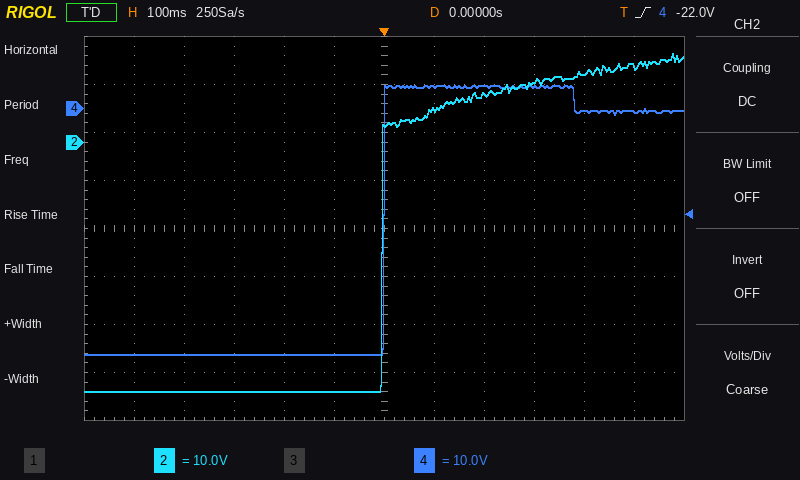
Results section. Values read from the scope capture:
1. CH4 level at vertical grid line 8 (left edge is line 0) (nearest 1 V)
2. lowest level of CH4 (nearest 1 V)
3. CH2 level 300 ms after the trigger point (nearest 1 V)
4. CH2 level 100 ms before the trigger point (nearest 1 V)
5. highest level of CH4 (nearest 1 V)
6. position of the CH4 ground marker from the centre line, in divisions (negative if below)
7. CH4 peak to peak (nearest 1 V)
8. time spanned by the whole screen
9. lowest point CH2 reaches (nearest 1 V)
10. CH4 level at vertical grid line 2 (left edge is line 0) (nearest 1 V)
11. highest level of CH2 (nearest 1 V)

5 V
-51 V
13 V
-52 V
5 V
+2.5 div
56 V
1.2 s
-52 V
-51 V
18 V
